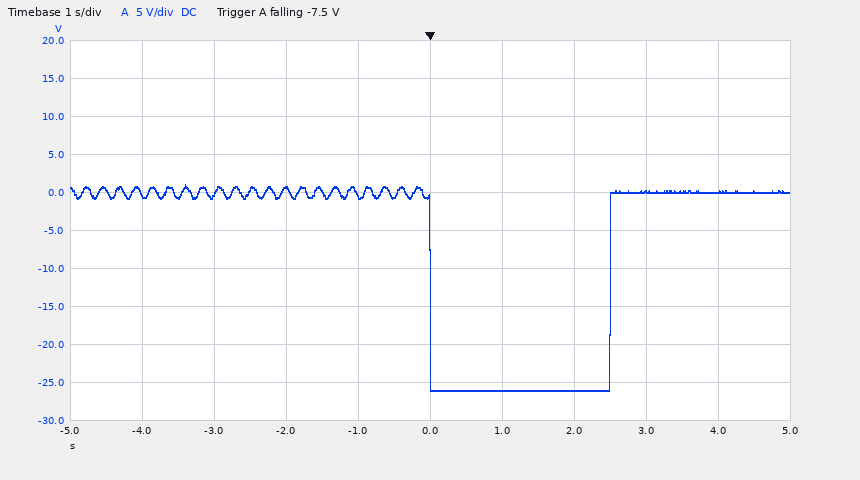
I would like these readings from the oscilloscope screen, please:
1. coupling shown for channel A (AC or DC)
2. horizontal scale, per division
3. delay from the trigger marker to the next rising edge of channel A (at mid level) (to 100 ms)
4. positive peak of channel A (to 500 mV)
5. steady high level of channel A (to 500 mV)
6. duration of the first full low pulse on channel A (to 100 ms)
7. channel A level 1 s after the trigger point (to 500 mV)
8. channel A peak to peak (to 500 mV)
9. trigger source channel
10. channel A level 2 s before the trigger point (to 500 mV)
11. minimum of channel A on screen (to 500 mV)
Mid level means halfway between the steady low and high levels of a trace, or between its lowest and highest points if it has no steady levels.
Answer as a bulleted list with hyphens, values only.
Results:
- DC
- 1 s
- 2.5 s
- 1.0 V
- 0.0 V
- 2.5 s
- -26.0 V
- 27.0 V
- channel A
- 500 mV
- -26.0 V
